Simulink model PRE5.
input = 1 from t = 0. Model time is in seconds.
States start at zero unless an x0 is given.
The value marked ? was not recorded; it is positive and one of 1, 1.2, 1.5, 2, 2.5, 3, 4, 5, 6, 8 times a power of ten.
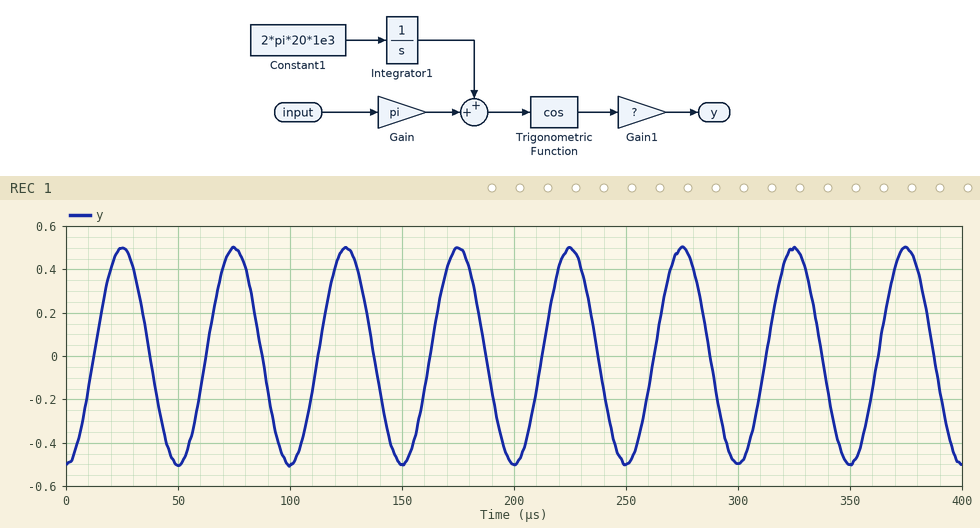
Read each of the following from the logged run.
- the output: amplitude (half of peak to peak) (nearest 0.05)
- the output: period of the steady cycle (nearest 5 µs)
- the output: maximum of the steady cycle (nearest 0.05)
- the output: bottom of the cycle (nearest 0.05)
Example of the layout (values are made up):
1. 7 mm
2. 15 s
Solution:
1. 0.50
2. 50 µs
3. 0.50
4. -0.50
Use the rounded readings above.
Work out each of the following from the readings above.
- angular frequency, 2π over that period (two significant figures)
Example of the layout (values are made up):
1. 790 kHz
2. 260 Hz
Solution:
1. 0.13 rad/µs
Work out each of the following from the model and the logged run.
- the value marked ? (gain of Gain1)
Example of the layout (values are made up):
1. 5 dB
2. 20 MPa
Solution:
1. 0.5
